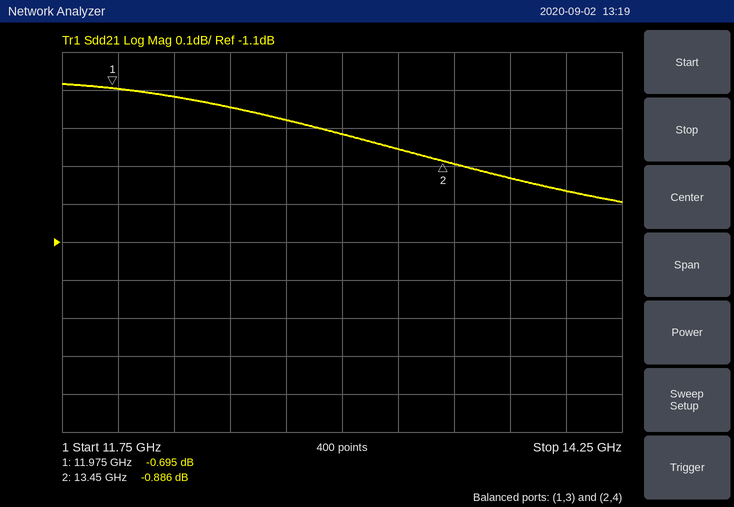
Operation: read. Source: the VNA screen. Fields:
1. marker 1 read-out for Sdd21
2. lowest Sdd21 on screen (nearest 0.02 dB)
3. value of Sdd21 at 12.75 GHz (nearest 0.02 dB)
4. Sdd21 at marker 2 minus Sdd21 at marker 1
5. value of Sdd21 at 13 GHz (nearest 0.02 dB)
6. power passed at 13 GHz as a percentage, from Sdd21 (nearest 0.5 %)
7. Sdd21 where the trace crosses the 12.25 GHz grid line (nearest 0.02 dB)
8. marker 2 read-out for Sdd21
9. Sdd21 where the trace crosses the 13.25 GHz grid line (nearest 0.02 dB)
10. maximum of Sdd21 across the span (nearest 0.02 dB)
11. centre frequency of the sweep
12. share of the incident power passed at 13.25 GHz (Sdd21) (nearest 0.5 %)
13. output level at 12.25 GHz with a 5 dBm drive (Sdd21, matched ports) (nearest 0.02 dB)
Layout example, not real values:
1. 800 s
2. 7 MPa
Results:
1. -0.695 dB
2. -1.00 dB
3. -0.78 dB
4. -0.191 dB
5. -0.82 dB
6. 83.0 %
7. -0.72 dB
8. -0.886 dB
9. -0.86 dB
10. -0.68 dB
11. 13 GHz
12. 82.0 %
13. 4.28 dBm
